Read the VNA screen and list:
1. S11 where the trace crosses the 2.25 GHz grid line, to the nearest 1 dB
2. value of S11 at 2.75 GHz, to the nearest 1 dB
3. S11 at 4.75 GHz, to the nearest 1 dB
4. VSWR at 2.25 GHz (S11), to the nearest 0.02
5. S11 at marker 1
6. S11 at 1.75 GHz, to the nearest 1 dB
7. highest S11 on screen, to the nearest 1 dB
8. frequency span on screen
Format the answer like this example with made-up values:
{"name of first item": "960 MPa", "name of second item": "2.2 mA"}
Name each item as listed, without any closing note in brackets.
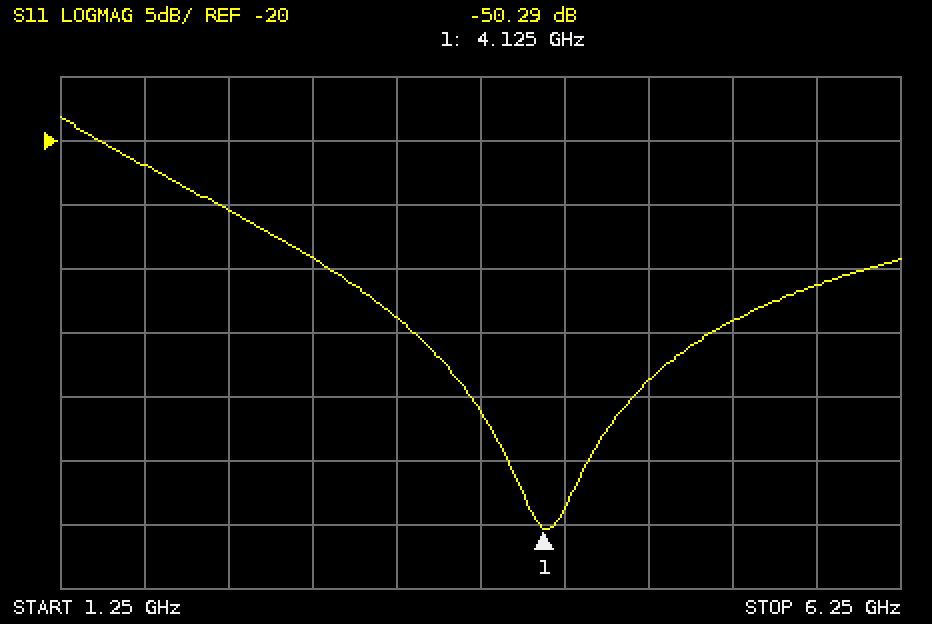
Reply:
{"S11 where the trace crosses the 2.25 GHz grid line, to the nearest 1 dB": "-25 dB", "value of S11 at 2.75 GHz, to the nearest 1 dB": "-29 dB", "S11 at 4.75 GHz, to the nearest 1 dB": "-39 dB", "VSWR at 2.25 GHz (S11), to the nearest 0.02": "1.12", "S11 at marker 1": "-50.29 dB", "S11 at 1.75 GHz, to the nearest 1 dB": "-22 dB", "highest S11 on screen, to the nearest 1 dB": "-18 dB", "frequency span on screen": "5 GHz"}
